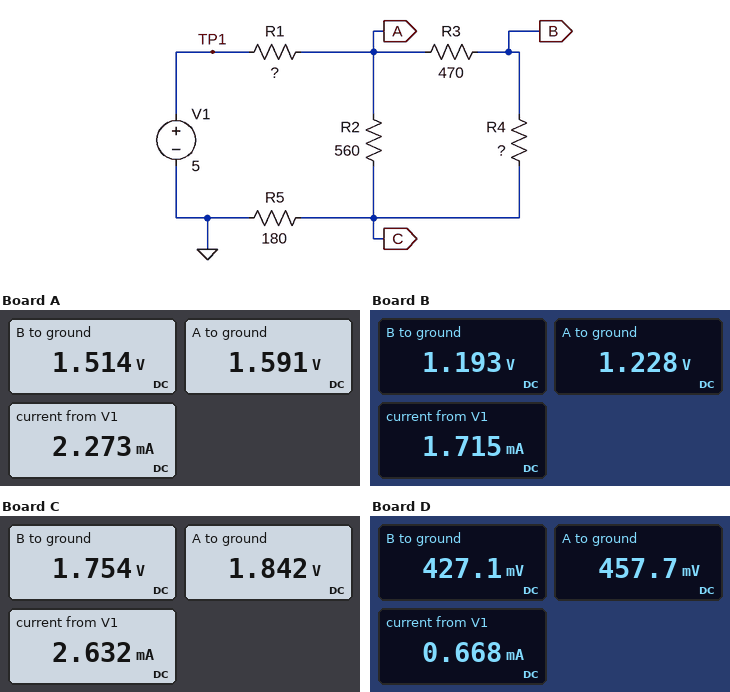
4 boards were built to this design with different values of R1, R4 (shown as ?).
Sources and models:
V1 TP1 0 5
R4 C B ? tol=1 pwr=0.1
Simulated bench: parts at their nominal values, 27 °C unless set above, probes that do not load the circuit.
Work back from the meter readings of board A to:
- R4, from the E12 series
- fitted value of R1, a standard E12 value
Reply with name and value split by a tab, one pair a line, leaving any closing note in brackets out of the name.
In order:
R4, from the E12 series	6.8 kΩ
fitted value of R1, a standard E12 value	1.5 kΩ
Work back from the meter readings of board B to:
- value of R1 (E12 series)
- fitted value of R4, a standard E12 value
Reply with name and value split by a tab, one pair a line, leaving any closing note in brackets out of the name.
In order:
value of R1	2.2 kΩ
fitted value of R4, a standard E12 value	12 kΩ
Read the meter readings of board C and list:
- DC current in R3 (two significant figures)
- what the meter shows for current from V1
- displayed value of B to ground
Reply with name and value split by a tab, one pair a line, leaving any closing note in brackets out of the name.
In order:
DC current in R3	190 µA
what the meter shows for current from V1	2.632 mA
displayed value of B to ground	1.754 V
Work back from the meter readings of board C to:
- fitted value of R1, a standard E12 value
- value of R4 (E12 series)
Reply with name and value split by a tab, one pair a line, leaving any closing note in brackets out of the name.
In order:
fitted value of R1, a standard E12 value	1.2 kΩ
value of R4	6.8 kΩ
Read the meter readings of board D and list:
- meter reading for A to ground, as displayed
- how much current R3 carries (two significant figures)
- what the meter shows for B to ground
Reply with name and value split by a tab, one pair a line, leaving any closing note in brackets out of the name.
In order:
meter reading for A to ground, as displayed	457.7 mV
how much current R3 carries	65 µA
what the meter shows for B to ground	427.1 mV
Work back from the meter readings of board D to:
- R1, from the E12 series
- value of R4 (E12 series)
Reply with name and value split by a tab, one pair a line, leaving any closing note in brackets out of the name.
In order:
R1, from the E12 series	6.8 kΩ
value of R4	4.7 kΩ
